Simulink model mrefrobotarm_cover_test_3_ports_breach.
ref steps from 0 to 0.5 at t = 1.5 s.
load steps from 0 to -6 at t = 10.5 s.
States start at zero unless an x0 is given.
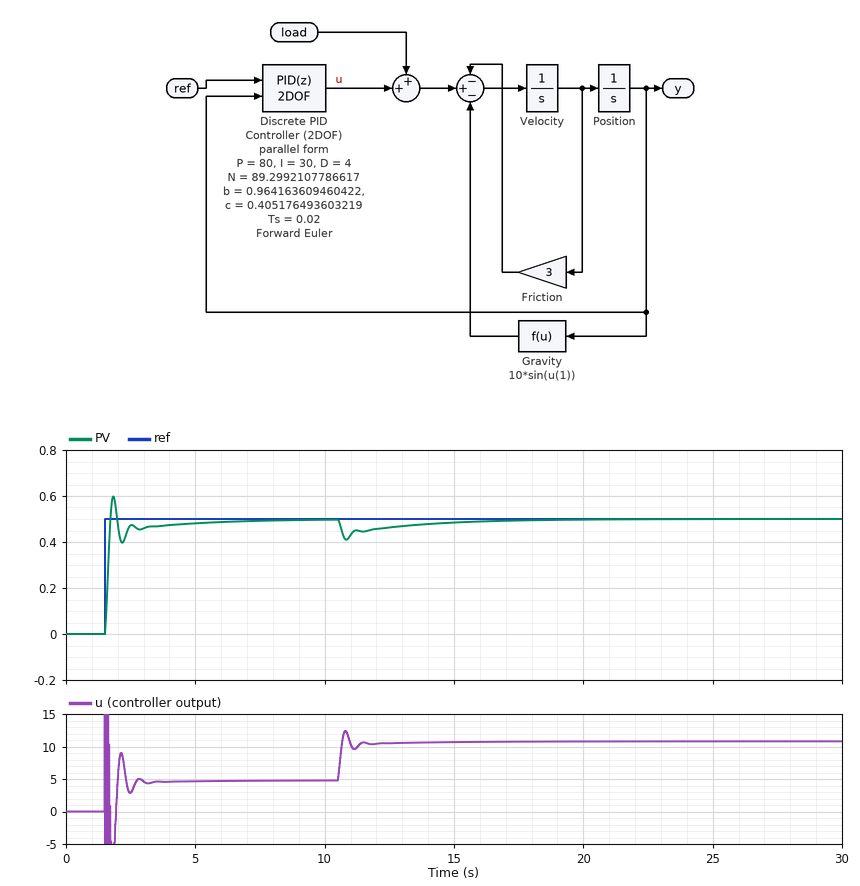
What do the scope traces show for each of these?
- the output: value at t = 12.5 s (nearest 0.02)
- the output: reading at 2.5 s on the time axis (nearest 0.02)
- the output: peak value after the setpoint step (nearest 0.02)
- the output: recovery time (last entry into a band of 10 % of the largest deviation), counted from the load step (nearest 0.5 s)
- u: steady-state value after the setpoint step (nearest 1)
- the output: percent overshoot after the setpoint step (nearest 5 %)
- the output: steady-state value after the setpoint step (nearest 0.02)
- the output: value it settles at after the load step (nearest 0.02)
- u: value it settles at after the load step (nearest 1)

0.46
0.48
0.60
6.0 s
5
20 %
0.50
0.50
11
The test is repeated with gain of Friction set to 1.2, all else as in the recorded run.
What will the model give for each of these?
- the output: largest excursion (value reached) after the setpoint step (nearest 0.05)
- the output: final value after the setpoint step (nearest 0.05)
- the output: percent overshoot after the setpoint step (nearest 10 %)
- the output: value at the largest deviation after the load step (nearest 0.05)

0.65
0.50
30 %
0.40
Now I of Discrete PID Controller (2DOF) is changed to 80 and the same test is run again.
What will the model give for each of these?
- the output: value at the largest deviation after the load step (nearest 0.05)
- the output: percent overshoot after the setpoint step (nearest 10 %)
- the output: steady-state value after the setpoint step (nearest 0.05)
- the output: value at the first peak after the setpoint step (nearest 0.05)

0.40
30 %
0.50
0.65
